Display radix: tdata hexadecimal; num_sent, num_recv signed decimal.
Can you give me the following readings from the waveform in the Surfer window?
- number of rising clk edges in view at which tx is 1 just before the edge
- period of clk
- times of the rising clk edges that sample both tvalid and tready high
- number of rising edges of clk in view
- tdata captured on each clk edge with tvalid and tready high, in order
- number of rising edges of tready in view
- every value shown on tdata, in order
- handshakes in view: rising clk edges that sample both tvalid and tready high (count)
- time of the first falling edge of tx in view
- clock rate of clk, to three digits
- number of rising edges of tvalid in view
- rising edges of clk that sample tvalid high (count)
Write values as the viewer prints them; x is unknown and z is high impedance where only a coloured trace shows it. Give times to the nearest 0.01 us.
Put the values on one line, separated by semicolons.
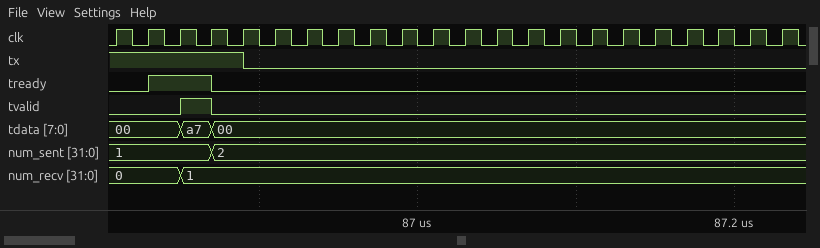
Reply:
5; 0.02 us; 86.87 us; 22; a7; 1; 00, a7, 00; 1; 86.89 us; 50.0 MHz; 1; 1
